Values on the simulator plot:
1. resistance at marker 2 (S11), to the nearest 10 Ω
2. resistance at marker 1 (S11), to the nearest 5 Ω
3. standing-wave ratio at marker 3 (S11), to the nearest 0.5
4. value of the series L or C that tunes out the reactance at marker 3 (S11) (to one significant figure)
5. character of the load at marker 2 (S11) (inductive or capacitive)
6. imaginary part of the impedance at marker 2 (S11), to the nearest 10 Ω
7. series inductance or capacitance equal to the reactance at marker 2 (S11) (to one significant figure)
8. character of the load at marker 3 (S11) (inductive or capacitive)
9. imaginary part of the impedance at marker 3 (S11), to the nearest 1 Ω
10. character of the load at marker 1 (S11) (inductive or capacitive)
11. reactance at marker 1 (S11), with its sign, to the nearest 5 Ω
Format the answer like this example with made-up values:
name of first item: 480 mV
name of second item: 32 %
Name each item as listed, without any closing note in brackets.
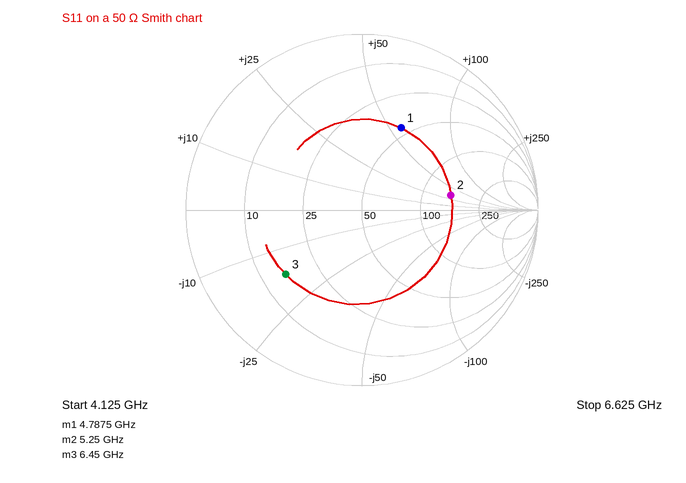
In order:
resistance at marker 2 (S11), to the nearest 10 Ω: 150 Ω
resistance at marker 1 (S11), to the nearest 5 Ω: 45 Ω
standing-wave ratio at marker 3 (S11), to the nearest 0.5: 3.5
value of the series L or C that tunes out the reactance at marker 3 (S11): 400 pH
character of the load at marker 2 (S11): inductive
imaginary part of the impedance at marker 2 (S11), to the nearest 10 Ω: +30 Ω
series inductance or capacitance equal to the reactance at marker 2 (S11): 1 nH
character of the load at marker 3 (S11): capacitive
imaginary part of the impedance at marker 3 (S11), to the nearest 1 Ω: -17 Ω
character of the load at marker 1 (S11): inductive
reactance at marker 1 (S11), with its sign, to the nearest 5 Ω: +55 Ω
